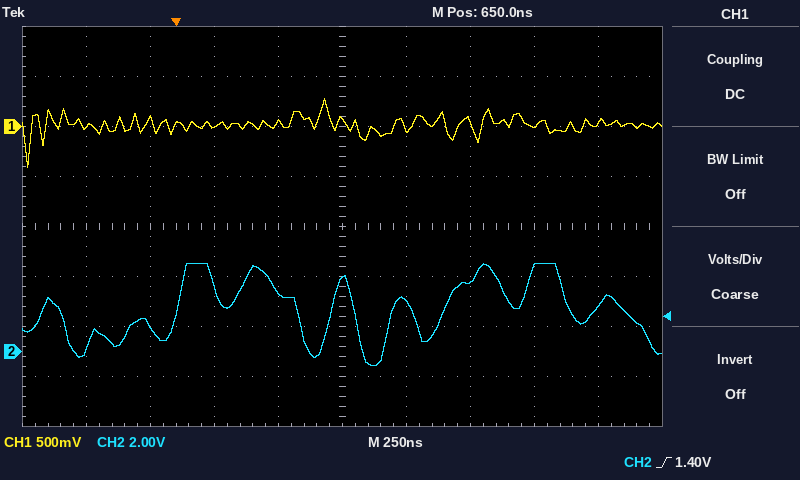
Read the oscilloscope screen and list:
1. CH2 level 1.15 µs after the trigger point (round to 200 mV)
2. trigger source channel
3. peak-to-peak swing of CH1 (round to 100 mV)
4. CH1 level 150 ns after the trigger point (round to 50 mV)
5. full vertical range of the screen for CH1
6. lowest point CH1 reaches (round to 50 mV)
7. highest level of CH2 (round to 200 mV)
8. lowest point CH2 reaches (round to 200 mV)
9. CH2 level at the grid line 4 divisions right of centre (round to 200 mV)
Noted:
2.8 V
CH2
700 mV
0 mV
4 V
-400 mV
3.6 V
-600 mV
1.8 V
